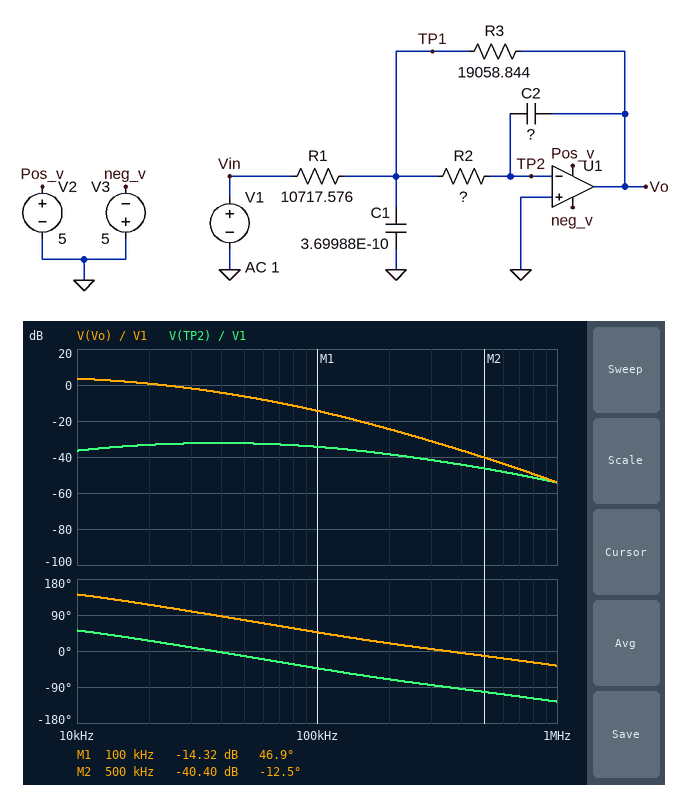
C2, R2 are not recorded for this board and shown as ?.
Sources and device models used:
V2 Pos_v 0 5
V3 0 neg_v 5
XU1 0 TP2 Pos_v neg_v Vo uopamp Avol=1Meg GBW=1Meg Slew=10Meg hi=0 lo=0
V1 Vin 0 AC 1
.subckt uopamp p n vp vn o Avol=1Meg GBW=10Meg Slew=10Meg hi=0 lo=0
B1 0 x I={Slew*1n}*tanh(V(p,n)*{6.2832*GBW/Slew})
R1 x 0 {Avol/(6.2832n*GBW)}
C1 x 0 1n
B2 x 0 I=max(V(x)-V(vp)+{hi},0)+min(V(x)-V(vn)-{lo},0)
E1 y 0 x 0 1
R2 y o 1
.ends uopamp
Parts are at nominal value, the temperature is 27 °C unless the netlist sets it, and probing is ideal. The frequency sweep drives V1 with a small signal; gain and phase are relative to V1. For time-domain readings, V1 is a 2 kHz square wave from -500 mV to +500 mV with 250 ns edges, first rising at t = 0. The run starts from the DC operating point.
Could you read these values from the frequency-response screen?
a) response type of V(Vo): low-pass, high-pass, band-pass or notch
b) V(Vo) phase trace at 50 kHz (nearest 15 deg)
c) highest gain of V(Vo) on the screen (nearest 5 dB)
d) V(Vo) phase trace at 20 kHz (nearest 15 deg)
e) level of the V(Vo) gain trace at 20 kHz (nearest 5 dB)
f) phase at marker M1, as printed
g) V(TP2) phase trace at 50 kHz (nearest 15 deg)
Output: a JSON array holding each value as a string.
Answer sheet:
["low-pass", "75 deg", "5 dB", "120 deg", "0 dB", "46.9 deg", "-15 deg"]
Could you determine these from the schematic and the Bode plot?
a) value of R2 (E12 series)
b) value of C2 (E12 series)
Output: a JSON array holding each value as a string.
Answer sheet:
["8.2 kΩ", "270 pF"]
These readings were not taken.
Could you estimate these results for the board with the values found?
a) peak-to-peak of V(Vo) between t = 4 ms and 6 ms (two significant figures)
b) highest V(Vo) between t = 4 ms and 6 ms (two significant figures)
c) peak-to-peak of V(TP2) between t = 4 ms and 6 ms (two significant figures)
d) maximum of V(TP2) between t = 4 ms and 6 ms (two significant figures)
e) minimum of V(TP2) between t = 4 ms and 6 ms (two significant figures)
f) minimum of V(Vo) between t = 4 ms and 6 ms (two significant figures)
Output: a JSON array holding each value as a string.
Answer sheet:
["1.8 V", "890 mV", "40 mV", "20 mV", "-20 mV", "-890 mV"]
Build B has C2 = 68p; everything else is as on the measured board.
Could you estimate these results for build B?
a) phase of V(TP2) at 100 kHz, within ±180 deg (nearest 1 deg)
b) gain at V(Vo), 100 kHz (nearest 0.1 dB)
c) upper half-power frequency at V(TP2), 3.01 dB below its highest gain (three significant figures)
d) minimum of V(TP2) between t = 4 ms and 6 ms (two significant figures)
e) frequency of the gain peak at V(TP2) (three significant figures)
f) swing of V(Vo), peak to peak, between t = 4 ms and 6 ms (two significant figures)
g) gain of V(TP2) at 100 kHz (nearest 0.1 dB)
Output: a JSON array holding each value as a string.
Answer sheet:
["-32 deg", "-2.0 dB", "134 kHz", "-58 mV", "70.2 kHz", "2.0 V", "-22.0 dB"]
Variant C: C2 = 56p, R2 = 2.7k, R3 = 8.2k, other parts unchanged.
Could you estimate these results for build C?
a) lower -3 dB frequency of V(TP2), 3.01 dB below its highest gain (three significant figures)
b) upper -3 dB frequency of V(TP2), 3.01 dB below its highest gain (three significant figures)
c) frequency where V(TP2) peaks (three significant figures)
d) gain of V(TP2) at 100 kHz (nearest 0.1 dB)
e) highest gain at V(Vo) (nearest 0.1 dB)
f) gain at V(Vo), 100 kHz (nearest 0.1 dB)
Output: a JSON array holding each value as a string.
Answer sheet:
["102 kHz", "251 kHz", "160 kHz", "-20.9 dB", "-0.7 dB", "-0.9 dB"]
